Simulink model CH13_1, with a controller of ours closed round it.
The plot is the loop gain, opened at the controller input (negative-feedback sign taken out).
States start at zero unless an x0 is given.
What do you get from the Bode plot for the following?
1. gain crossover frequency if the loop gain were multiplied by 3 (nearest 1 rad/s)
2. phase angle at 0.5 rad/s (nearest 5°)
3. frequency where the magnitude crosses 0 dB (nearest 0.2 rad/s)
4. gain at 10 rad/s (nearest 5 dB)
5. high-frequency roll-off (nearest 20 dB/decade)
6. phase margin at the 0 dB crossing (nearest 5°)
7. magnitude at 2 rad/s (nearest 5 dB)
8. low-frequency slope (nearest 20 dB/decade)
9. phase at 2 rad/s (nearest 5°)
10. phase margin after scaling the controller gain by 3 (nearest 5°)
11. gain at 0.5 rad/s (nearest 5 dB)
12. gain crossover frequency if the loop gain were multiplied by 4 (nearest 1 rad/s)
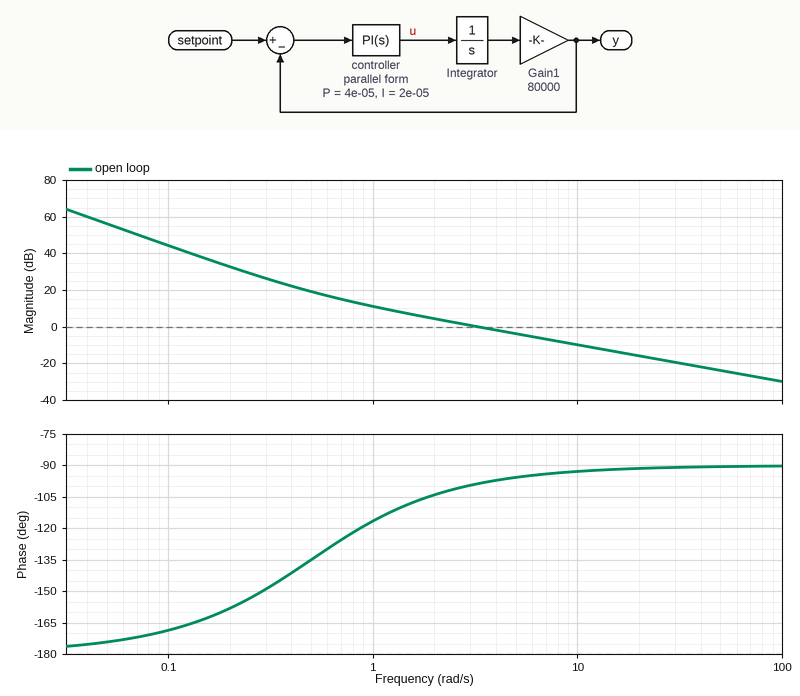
10 rad/s
-135°
3.2 rad/s
-10 dB
-20 dB/decade
80°
5 dB
-40 dB/decade
-105°
85°
20 dB
13 rad/s
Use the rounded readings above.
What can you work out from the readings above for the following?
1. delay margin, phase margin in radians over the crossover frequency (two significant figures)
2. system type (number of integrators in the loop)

0.44 s
2
